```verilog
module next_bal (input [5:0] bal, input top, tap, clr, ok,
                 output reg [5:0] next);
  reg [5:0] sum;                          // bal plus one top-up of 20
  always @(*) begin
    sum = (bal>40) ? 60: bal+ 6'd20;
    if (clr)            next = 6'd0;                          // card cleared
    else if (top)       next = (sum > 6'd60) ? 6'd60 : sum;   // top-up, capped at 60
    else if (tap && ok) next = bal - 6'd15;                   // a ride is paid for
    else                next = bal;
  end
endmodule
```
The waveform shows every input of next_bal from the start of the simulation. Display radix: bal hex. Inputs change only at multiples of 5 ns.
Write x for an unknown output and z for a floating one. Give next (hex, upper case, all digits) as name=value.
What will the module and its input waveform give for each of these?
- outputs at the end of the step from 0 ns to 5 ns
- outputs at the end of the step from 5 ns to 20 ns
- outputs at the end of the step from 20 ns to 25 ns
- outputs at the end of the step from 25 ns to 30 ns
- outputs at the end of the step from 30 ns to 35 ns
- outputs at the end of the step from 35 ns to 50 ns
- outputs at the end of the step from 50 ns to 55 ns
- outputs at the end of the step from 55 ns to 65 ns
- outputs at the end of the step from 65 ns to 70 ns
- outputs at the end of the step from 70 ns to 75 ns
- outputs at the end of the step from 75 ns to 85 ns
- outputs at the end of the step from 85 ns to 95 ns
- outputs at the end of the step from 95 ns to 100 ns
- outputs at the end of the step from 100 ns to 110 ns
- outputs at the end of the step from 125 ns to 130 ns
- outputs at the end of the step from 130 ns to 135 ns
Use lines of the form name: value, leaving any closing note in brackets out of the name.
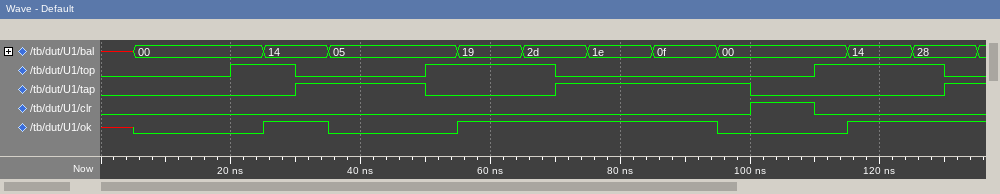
outputs at the end of the step from 0 ns to 5 ns: next=x
outputs at the end of the step from 5 ns to 20 ns: next=00
outputs at the end of the step from 20 ns to 25 ns: next=14
outputs at the end of the step from 25 ns to 30 ns: next=28
outputs at the end of the step from 30 ns to 35 ns: next=05
outputs at the end of the step from 35 ns to 50 ns: next=05
outputs at the end of the step from 50 ns to 55 ns: next=19
outputs at the end of the step from 55 ns to 65 ns: next=2D
outputs at the end of the step from 65 ns to 70 ns: next=3C
outputs at the end of the step from 70 ns to 75 ns: next=1E
outputs at the end of the step from 75 ns to 85 ns: next=0F
outputs at the end of the step from 85 ns to 95 ns: next=00
outputs at the end of the step from 95 ns to 100 ns: next=00
outputs at the end of the step from 100 ns to 110 ns: next=00
outputs at the end of the step from 125 ns to 130 ns: next=3C
outputs at the end of the step from 130 ns to 135 ns: next=19
